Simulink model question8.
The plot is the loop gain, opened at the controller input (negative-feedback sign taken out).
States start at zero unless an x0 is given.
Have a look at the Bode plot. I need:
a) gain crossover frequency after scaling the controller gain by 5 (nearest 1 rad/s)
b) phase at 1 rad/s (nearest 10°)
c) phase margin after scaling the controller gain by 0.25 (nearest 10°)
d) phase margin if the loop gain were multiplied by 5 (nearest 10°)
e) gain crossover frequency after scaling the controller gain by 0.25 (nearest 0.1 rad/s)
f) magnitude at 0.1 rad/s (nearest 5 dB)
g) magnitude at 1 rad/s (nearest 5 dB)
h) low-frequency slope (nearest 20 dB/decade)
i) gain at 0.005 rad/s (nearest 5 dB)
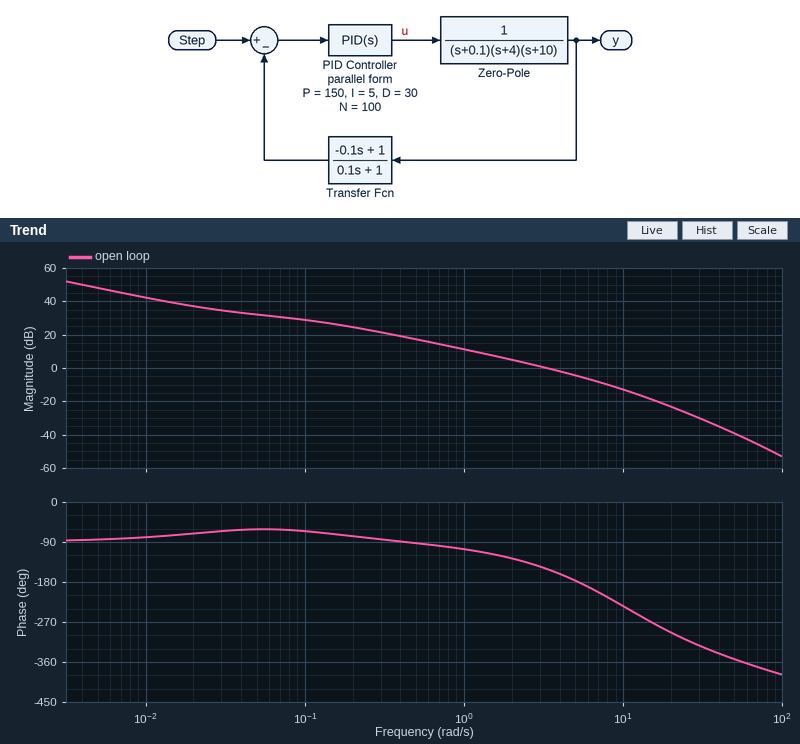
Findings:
11 rad/s
-110°
80°
-60°
0.9 rad/s
30 dB
10 dB
-20 dB/decade
50 dB
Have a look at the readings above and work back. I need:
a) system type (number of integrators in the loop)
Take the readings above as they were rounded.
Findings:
1
